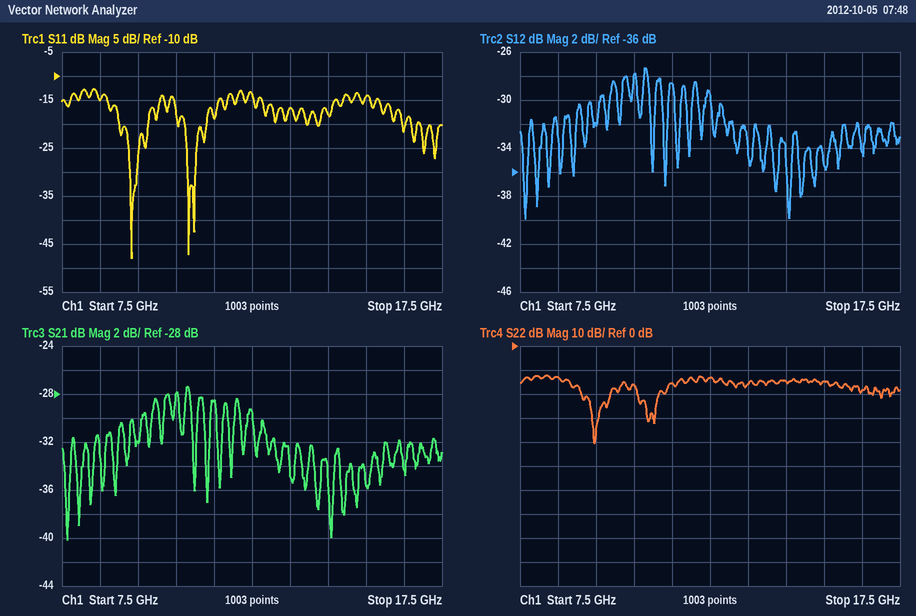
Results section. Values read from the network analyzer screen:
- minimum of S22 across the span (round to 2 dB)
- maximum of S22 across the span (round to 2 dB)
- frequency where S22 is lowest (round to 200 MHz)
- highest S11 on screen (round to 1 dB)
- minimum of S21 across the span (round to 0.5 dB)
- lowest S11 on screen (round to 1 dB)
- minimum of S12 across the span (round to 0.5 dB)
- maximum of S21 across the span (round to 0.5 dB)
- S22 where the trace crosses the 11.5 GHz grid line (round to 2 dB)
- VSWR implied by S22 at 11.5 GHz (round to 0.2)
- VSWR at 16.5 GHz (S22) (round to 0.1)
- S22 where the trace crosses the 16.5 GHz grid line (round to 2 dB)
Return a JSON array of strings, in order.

["-40 dB", "-12 dB", "9.4 GHz", "-13 dB", "-40.0 dB", "-48 dB", "-40.0 dB", "-27.5 dB", "-16 dB", "1.4", "1.3", "-18 dB"]
